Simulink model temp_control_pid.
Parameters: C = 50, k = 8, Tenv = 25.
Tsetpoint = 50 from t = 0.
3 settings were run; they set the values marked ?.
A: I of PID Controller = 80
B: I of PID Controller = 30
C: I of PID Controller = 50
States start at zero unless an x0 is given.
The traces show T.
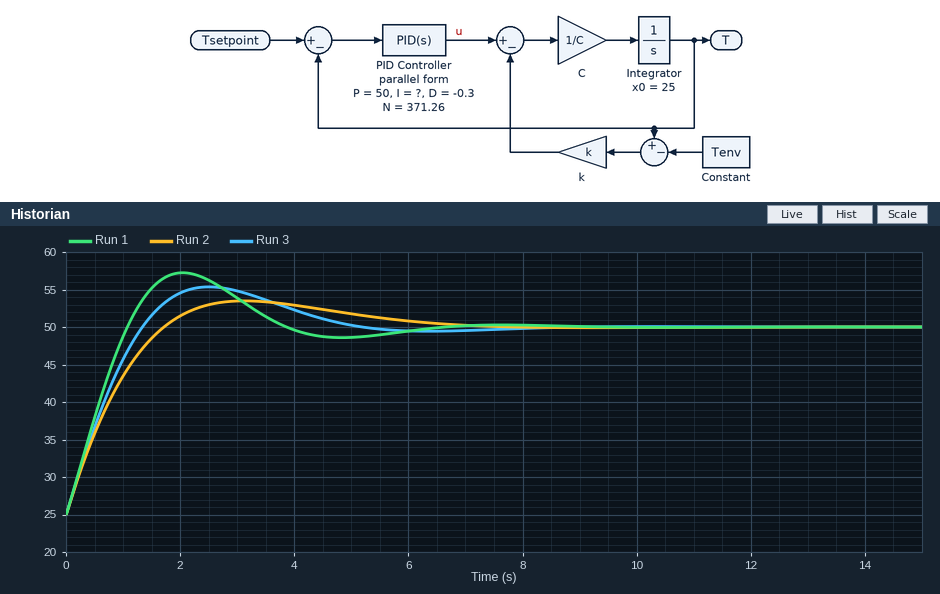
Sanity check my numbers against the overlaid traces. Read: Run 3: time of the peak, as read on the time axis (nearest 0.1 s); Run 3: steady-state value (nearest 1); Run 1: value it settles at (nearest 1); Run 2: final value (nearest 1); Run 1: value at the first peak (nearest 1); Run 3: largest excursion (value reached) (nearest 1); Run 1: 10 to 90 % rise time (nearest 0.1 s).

2.5 s
50
50
50
57
55
0.8 s
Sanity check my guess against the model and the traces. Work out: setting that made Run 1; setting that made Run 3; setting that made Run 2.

A
C
B
